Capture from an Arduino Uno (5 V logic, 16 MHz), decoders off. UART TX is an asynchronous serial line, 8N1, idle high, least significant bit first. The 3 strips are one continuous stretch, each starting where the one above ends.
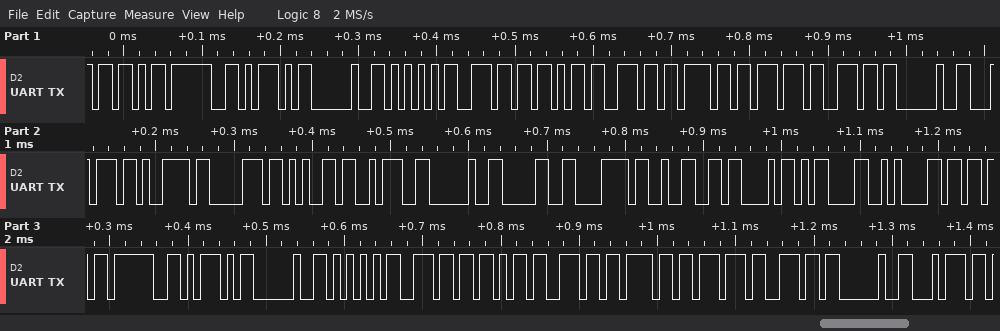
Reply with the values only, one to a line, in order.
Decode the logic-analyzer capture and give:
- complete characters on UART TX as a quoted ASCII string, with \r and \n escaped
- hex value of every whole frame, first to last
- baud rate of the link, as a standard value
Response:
"[?] Unknown type: 0x2C\r\n[?] Unknown t"
5B 3F 5D 20 55 6E 6B 6E 6F 77 6E 20 74 79 70 65 3A 20 30 78 32 43 0D 0A 5B 3F 5D 20 55 6E 6B 6E 6F 77 6E 20 74
115200 baud
